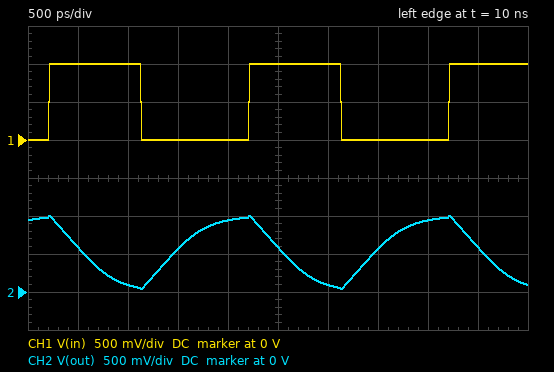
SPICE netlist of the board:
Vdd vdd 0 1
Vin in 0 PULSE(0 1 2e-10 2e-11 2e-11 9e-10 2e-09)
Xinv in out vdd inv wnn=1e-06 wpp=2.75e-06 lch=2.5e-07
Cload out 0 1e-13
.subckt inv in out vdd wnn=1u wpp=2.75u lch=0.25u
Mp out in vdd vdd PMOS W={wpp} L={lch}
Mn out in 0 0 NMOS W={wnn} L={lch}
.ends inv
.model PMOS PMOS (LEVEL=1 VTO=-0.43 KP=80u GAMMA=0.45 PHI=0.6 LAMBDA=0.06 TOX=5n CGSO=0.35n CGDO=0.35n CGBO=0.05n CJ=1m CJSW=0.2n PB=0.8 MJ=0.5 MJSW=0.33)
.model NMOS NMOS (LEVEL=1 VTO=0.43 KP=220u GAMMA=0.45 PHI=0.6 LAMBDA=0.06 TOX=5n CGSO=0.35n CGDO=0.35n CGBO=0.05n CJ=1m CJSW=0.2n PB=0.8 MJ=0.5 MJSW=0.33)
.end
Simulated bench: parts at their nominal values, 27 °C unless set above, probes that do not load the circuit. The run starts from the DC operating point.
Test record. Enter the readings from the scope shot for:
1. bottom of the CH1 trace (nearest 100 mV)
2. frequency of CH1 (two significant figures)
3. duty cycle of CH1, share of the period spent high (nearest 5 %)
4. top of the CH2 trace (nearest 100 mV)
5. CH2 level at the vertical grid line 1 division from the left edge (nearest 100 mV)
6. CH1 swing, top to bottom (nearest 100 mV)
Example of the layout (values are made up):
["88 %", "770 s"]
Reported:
["0 V", "500 MHz", "45 %", "1.0 V", "600 mV", "1.0 V"]
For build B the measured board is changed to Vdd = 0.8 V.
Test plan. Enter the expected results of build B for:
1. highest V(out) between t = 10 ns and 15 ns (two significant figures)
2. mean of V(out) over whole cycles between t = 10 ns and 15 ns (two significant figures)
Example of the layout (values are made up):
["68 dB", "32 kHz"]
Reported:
["640 mV", "270 mV"]
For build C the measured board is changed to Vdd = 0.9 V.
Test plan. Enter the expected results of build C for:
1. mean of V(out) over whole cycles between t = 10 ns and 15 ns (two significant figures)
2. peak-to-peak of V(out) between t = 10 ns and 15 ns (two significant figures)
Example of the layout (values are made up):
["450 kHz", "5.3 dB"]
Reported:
["420 mV", "840 mV"]
